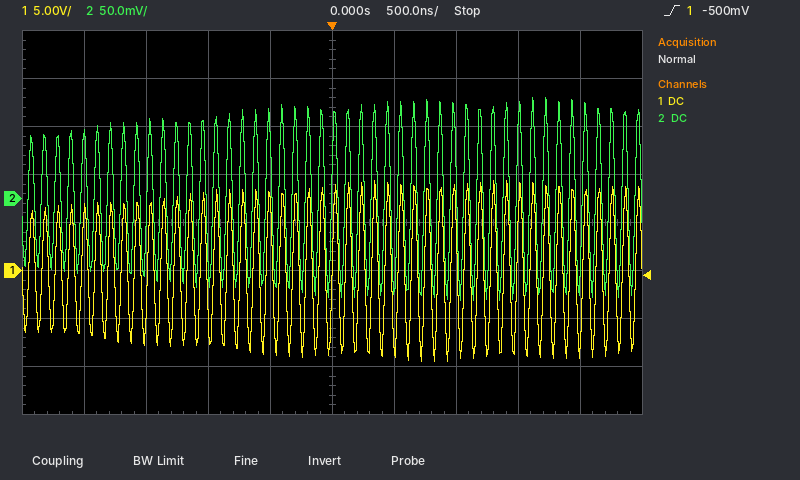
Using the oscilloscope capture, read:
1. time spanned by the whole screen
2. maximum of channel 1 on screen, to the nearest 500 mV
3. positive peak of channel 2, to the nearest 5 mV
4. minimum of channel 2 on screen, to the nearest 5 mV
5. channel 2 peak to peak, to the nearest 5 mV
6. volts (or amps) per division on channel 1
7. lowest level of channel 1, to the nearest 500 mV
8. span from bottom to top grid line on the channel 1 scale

5 µs
9.5 V
105 mV
-105 mV
210 mV
5 V
-9.5 V
40 V
